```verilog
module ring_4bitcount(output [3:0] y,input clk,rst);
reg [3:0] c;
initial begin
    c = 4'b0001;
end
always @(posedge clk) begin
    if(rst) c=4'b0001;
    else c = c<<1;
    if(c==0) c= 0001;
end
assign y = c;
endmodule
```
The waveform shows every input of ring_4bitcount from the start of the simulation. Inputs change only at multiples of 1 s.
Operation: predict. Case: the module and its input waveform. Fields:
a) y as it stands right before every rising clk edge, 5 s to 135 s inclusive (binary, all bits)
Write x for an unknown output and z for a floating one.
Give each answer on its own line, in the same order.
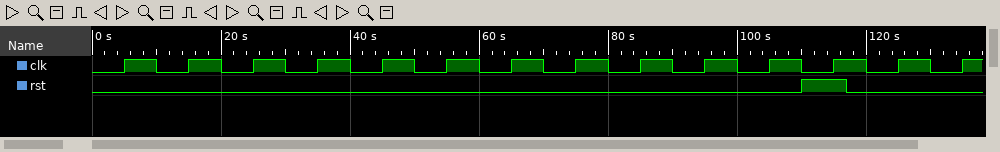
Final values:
0001, 0010, 0100, 1000, 0001, 0010, 0100, 1000, 0001, 0010, 0100, 1000, 0001, 0010
